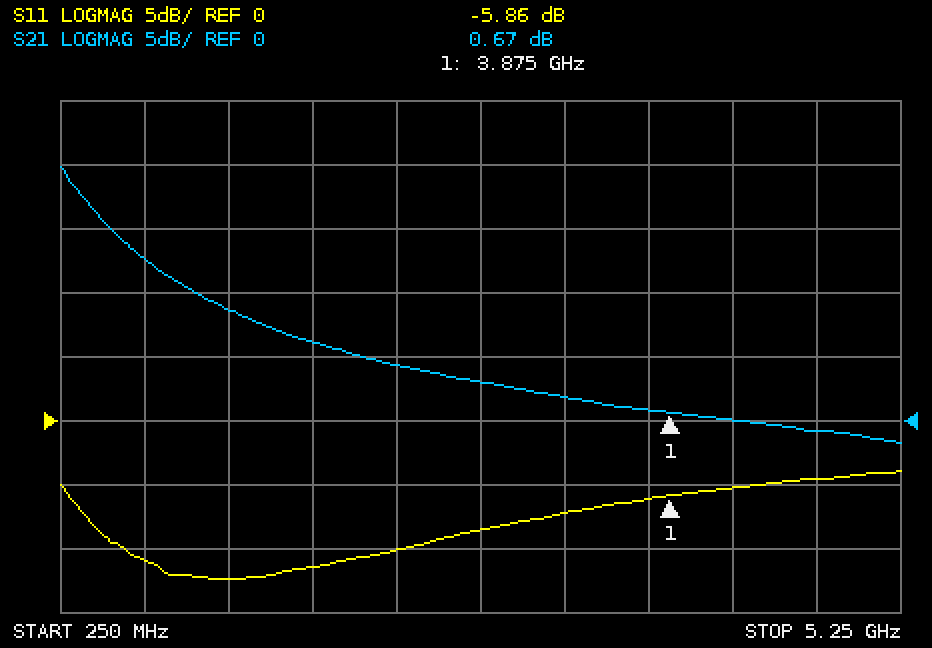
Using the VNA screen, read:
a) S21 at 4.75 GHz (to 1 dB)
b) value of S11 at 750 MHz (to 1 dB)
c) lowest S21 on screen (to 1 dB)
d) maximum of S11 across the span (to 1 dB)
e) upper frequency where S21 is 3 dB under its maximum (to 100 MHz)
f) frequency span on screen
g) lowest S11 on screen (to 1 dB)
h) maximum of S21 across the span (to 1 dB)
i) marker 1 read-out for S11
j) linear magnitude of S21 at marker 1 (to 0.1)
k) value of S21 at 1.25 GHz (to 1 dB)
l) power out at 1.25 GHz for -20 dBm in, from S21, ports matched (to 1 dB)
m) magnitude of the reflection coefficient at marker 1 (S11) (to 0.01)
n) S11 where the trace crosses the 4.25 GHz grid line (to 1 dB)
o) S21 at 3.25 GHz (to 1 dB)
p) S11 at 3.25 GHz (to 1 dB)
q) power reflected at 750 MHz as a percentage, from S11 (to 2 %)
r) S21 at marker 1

-1 dB
-11 dB
-2 dB
-4 dB
400 MHz
5 GHz
-12 dB
20 dB
-5.86 dB
1.1
9 dB
-11 dBm
0.51
-5 dB
2 dB
-7 dB
8 %
0.67 dB
